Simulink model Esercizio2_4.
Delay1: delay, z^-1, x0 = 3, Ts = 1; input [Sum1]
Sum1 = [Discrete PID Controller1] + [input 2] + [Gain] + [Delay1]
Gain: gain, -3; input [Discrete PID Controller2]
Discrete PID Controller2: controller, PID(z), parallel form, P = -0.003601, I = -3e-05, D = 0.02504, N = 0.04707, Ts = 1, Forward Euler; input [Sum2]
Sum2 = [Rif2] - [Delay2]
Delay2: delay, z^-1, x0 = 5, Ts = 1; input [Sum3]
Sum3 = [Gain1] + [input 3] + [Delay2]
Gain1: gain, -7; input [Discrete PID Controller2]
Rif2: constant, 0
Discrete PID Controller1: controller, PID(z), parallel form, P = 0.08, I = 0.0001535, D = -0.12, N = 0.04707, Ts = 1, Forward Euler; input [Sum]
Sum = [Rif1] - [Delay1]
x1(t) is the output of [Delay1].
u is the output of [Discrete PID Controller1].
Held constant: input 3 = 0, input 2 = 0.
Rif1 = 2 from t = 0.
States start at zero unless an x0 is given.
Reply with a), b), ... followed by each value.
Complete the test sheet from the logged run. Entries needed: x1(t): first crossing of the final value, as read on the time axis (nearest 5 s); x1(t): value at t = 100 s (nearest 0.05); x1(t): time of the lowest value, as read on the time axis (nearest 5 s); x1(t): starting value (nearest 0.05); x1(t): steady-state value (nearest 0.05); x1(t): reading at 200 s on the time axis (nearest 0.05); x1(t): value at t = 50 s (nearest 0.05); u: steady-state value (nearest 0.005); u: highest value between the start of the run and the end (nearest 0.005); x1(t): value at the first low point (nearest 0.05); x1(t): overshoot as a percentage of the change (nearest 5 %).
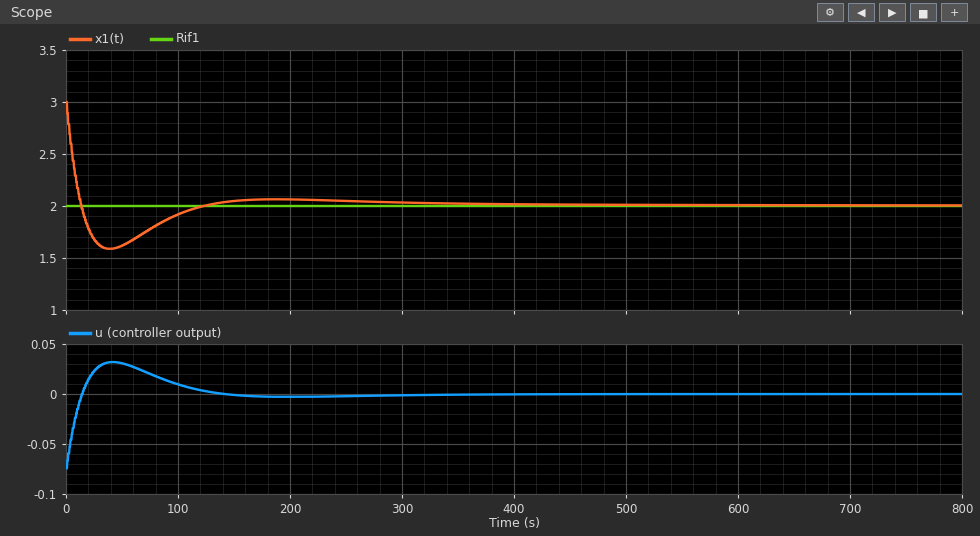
a) 15 s
b) 1.90
c) 40 s
d) 3.00
e) 2.00
f) 2.05
g) 1.60
h) 0.000
i) 0.030
j) 1.60
k) 40 %
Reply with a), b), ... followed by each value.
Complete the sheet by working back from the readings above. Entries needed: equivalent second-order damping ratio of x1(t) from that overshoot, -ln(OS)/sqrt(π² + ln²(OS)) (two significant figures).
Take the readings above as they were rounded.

a) 0.28
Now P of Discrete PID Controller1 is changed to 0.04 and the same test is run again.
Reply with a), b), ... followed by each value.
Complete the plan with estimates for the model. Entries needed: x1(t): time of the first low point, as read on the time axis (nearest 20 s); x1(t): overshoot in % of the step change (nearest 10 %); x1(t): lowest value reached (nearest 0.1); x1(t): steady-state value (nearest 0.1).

a) 60 s
b) 60 %
c) 1.4
d) 2.0
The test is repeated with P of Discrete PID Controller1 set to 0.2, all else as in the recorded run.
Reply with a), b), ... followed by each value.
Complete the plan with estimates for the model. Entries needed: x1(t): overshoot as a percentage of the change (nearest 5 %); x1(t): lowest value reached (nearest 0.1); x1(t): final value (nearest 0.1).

a) 20 %
b) 1.8
c) 2.0
